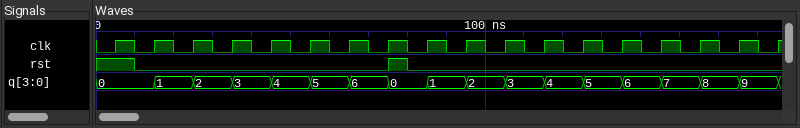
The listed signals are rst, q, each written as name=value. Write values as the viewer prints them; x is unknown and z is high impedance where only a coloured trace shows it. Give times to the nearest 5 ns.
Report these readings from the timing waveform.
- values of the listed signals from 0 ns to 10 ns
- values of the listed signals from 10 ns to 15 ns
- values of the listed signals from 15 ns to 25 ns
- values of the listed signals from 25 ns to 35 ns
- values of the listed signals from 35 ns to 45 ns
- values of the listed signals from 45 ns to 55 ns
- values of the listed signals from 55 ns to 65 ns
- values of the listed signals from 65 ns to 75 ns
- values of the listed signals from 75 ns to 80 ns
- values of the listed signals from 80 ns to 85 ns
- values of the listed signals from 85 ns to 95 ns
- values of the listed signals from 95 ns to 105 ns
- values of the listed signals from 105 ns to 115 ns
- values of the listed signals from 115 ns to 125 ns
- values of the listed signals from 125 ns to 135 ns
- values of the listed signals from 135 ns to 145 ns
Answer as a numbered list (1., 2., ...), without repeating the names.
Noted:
1. rst=1, q=0
2. rst=0, q=0
3. rst=0, q=1
4. rst=0, q=2
5. rst=0, q=3
6. rst=0, q=4
7. rst=0, q=5
8. rst=0, q=6
9. rst=1, q=0
10. rst=0, q=0
11. rst=0, q=1
12. rst=0, q=2
13. rst=0, q=3
14. rst=0, q=4
15. rst=0, q=5
16. rst=0, q=6
